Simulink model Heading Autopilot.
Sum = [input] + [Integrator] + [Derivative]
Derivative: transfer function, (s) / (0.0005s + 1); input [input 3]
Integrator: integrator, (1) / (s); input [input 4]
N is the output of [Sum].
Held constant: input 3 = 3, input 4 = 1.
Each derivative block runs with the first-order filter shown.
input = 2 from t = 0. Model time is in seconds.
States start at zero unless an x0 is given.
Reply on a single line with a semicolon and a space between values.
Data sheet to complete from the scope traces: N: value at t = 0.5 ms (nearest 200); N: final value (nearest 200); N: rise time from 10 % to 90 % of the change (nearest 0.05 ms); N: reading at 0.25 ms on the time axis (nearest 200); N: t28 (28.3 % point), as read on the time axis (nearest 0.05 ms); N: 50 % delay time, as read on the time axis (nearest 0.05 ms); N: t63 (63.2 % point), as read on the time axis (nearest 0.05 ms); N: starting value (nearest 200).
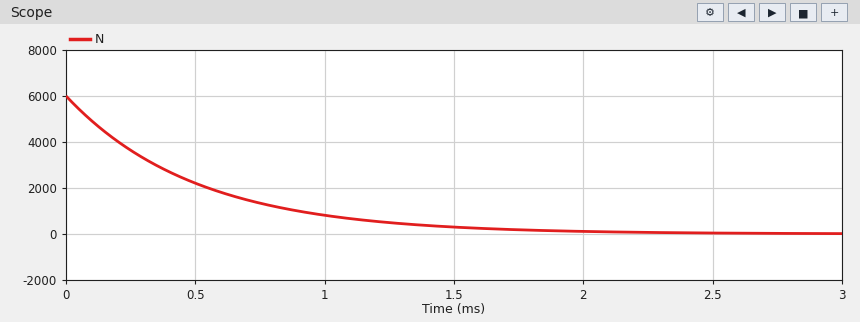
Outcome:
2200; 0; 1.10 ms; 3600; 0.15 ms; 0.35 ms; 0.50 ms; 6000
